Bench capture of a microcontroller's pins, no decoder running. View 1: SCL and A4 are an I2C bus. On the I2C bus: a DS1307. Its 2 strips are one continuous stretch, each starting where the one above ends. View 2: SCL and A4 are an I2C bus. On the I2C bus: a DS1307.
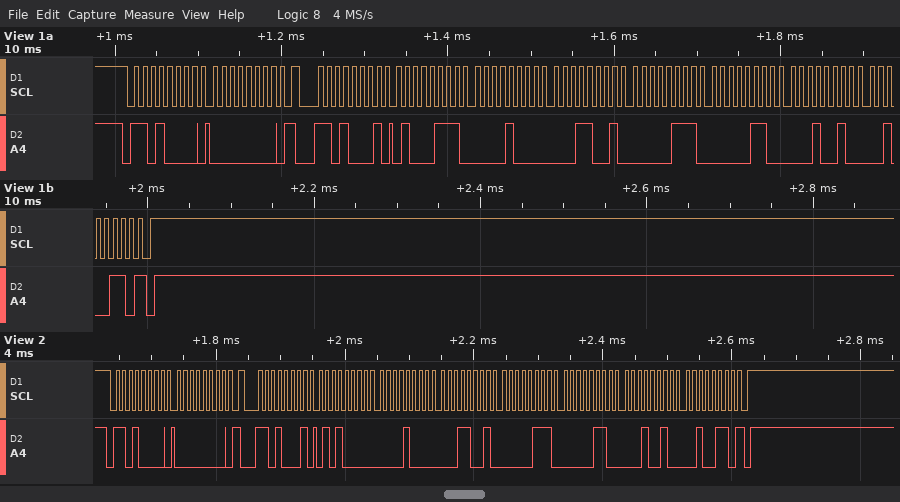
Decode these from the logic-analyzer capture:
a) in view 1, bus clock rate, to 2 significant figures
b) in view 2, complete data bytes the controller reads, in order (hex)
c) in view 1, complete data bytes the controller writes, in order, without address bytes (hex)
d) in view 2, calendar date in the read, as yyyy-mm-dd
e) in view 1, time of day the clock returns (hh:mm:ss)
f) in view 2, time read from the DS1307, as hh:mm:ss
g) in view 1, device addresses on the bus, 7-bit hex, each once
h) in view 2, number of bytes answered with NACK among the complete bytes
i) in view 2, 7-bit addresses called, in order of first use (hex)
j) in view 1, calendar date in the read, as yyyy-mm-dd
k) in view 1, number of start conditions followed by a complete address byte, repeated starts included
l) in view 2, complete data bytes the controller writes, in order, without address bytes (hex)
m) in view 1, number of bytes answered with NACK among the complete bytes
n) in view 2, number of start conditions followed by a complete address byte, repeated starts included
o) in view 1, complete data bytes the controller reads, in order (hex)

100 kHz
50 08 19 07 06 12 26
00
2026-12-06
19:08:47
19:08:50
0x68
1
0x68
2026-12-06
2
00
1
2
47 08 19 07 06 12 26
